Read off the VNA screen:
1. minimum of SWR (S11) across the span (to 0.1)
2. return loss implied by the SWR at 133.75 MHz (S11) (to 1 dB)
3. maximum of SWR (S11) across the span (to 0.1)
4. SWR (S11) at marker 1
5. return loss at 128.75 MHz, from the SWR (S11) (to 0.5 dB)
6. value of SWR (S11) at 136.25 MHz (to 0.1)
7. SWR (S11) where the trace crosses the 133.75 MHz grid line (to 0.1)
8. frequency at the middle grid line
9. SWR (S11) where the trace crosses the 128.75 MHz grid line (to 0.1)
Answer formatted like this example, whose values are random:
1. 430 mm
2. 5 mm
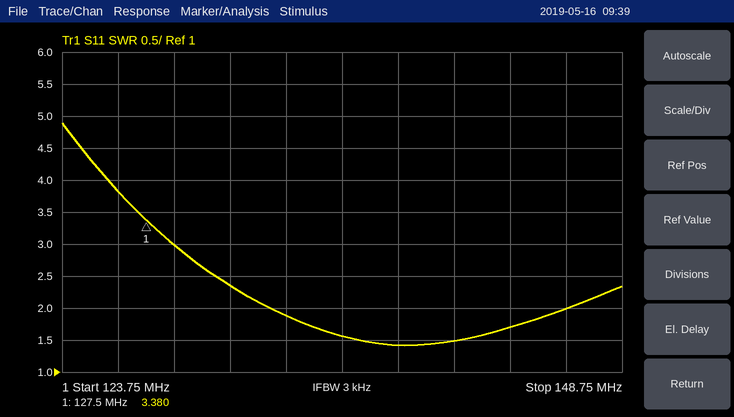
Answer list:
1. 1.4
2. 10 dB
3. 4.9
4. 3.380
5. 6.0 dB
6. 1.6
7. 1.9
8. 136.25 MHz
9. 3.0
